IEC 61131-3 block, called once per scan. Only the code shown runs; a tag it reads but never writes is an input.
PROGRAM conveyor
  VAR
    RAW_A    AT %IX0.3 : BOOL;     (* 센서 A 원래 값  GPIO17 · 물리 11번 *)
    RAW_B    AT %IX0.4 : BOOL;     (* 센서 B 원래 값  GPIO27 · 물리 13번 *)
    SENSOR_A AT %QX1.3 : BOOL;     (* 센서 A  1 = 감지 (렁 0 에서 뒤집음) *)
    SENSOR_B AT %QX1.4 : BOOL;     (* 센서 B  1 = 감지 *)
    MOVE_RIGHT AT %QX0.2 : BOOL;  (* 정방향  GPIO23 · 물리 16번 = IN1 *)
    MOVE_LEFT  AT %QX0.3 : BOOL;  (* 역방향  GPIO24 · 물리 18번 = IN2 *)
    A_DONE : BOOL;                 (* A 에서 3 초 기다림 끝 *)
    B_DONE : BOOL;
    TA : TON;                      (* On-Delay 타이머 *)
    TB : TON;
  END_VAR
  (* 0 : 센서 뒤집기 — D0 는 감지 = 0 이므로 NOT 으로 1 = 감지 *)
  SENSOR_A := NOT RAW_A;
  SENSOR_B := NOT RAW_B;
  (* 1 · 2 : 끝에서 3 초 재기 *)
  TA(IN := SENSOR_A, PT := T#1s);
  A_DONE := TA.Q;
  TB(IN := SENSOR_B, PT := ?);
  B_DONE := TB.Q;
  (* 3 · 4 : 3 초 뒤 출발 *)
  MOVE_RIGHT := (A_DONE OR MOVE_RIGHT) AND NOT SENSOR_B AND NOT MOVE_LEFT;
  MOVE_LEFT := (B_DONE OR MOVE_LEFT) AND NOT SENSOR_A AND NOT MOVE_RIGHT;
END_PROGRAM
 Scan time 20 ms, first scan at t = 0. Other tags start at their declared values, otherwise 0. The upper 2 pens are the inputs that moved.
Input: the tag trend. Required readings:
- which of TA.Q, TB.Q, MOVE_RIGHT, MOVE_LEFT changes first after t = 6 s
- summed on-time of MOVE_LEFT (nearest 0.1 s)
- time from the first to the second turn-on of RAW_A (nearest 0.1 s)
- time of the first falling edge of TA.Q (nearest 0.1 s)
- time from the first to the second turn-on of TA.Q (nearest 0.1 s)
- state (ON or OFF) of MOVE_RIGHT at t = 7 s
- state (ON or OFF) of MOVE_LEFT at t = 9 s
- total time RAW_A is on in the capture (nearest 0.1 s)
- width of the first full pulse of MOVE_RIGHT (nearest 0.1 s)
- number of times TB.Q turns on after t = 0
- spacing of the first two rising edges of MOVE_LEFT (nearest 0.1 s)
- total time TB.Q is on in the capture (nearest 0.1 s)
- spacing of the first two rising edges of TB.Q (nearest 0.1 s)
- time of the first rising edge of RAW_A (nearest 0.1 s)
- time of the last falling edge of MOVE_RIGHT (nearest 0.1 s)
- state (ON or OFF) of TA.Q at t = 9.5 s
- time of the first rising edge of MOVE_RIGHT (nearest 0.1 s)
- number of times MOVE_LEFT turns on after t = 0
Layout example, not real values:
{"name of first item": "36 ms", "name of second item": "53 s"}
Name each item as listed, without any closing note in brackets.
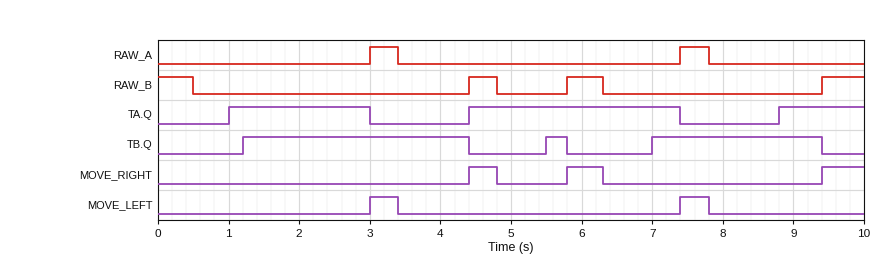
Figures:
{"which of TA.Q, TB.Q, MOVE_RIGHT, MOVE_LEFT changes first after t = 6 s": "MOVE_RIGHT", "summed on-time of MOVE_LEFT": "0.8 s", "time from the first to the second turn-on of RAW_A": "4.4 s", "time of the first falling edge of TA.Q": "3.0 s", "time from the first to the second turn-on of TA.Q": "3.4 s", "state (ON or OFF) of MOVE_RIGHT at t = 7 s": "OFF", "state (ON or OFF) of MOVE_LEFT at t = 9 s": "OFF", "total time RAW_A is on in the capture": "0.8 s", "width of the first full pulse of MOVE_RIGHT": "0.4 s", "number of times TB.Q turns on after t = 0": "3", "spacing of the first two rising edges of MOVE_LEFT": "4.4 s", "total time TB.Q is on in the capture": "5.9 s", "spacing of the first two rising edges of TB.Q": "4.3 s", "time of the first rising edge of RAW_A": "3.0 s", "time of the last falling edge of MOVE_RIGHT": "6.3 s", "state (ON or OFF) of TA.Q at t = 9.5 s": "ON", "time of the first rising edge of MOVE_RIGHT": "4.4 s", "number of times MOVE_LEFT turns on after t = 0": "2"}
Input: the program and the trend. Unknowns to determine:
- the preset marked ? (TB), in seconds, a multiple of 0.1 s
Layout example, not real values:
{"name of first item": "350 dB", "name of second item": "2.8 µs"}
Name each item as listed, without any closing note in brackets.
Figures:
{"the preset marked ? (TB), in seconds, a multiple of 0.1 s": "0.7 s"}
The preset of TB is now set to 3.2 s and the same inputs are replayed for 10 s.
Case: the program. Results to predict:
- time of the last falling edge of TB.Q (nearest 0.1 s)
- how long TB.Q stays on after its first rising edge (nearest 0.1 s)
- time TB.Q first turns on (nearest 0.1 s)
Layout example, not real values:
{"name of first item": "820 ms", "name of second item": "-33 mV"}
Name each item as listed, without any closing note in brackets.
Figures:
{"time of the last falling edge of TB.Q": "4.4 s", "how long TB.Q stays on after its first rising edge": "0.7 s", "time TB.Q first turns on": "3.7 s"}
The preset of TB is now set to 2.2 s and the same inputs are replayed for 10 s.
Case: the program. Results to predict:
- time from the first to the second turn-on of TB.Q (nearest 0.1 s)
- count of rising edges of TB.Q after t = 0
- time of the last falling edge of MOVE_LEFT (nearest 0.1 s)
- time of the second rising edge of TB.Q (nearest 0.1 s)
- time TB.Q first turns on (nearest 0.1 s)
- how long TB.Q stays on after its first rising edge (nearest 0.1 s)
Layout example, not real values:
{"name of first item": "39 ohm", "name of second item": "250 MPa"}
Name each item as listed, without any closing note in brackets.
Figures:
{"time from the first to the second turn-on of TB.Q": "5.8 s", "count of rising edges of TB.Q after t = 0": "2", "time of the last falling edge of MOVE_LEFT": "3.4 s", "time of the second rising edge of TB.Q": "8.5 s", "time TB.Q first turns on": "2.7 s", "how long TB.Q stays on after its first rising edge": "1.7 s"}
